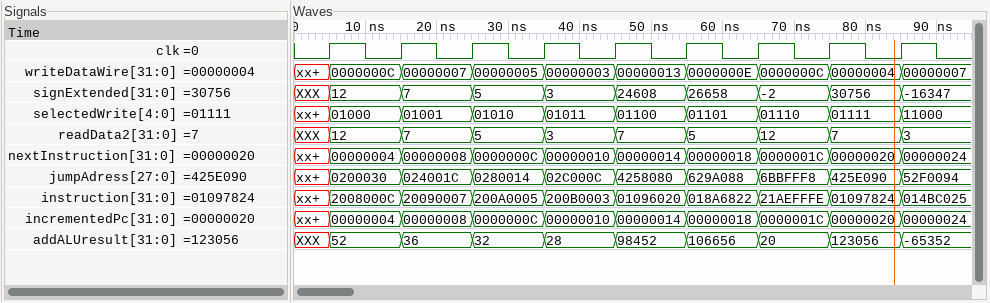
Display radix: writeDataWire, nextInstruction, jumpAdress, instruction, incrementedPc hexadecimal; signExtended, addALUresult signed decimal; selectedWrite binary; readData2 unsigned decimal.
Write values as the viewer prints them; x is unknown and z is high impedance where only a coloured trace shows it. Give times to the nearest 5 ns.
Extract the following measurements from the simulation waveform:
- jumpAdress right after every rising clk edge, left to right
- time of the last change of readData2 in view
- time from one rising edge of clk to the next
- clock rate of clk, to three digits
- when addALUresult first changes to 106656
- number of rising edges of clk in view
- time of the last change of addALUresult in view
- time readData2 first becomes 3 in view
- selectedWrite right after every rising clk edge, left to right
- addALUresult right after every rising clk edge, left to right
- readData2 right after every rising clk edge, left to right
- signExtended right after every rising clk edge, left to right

0200030, 024001C, 0280014, 02C000C, 4258080, 629A088, 6BBFFF8, 425E090, 52F0094
85 ns
10 ns
100 MHz
55 ns
9
85 ns
35 ns
01000, 01001, 01010, 01011, 01100, 01101, 01110, 01111, 11000
52, 36, 32, 28, 98452, 106656, 20, 123056, -65352
12, 7, 5, 3, 7, 5, 12, 7, 3
12, 7, 5, 3, 24608, 26658, -2, 30756, -16347
